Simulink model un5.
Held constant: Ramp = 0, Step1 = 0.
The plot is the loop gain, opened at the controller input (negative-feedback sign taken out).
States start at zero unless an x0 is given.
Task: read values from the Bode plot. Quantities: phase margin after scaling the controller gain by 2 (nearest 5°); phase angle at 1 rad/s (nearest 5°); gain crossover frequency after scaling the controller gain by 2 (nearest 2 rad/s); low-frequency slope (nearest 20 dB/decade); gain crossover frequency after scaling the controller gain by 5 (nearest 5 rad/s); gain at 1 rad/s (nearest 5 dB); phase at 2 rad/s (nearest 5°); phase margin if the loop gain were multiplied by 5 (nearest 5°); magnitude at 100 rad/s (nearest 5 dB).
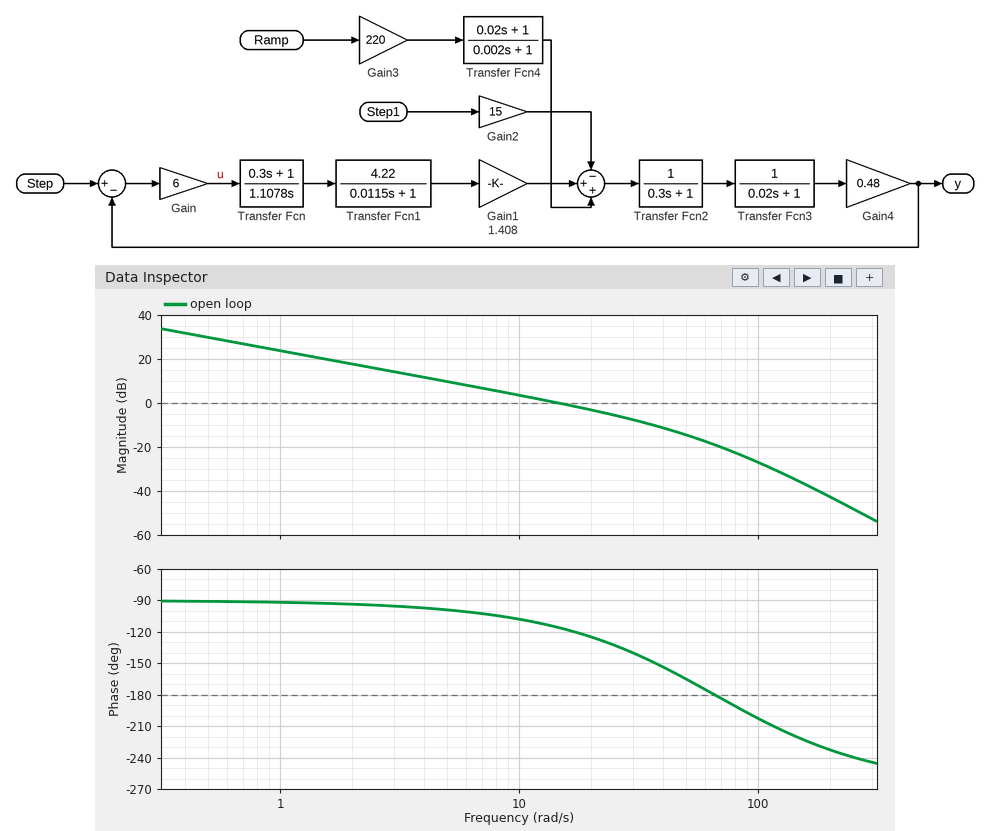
45°
-90°
26 rad/s
-20 dB/decade
50 rad/s
25 dB
-95°
15°
-25 dB
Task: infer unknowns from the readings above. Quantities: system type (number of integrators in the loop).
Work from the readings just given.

1
